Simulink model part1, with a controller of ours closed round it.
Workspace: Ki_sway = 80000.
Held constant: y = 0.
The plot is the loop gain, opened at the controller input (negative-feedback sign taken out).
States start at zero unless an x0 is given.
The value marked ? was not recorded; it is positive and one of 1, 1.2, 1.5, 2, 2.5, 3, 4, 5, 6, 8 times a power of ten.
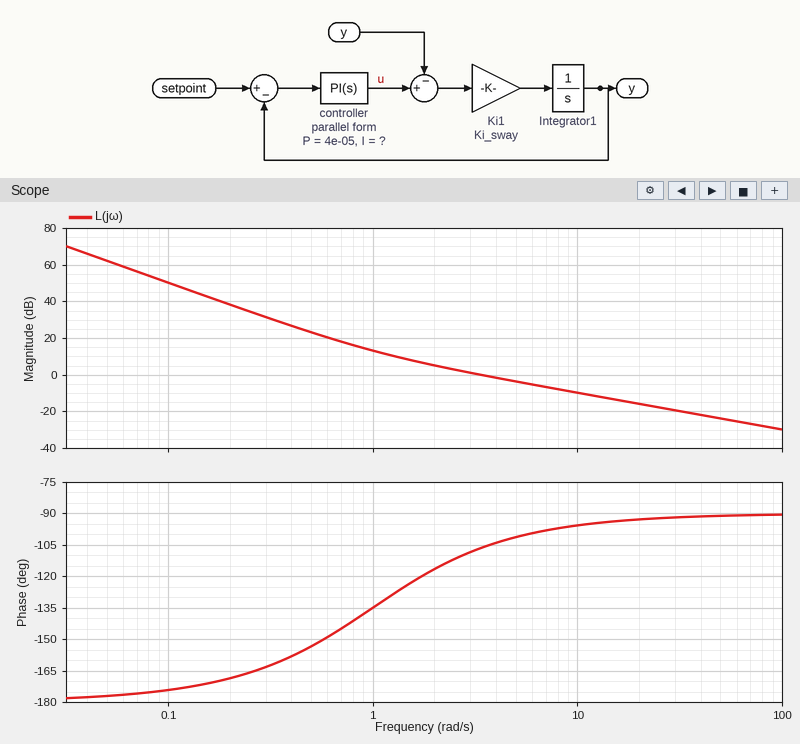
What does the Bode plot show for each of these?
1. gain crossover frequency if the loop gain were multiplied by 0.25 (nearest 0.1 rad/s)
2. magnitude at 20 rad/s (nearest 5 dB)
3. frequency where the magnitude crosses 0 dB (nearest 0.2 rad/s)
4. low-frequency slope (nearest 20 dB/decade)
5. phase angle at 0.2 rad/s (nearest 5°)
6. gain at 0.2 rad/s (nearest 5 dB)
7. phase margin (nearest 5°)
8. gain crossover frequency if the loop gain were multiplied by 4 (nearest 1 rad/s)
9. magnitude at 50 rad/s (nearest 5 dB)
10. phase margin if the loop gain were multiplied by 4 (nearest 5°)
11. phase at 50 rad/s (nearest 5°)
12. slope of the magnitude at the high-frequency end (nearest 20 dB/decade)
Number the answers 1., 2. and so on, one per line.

1. 1.1 rad/s
2. -15 dB
3. 3.4 rad/s
4. -40 dB/decade
5. -170°
6. 40 dB
7. 75°
8. 13 rad/s
9. -25 dB
10. 85°
11. -90°
12. -20 dB/decade
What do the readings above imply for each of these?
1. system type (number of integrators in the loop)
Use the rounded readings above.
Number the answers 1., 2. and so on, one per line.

1. 2
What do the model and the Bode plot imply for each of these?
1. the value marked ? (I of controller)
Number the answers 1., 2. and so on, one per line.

1. 4e-05
